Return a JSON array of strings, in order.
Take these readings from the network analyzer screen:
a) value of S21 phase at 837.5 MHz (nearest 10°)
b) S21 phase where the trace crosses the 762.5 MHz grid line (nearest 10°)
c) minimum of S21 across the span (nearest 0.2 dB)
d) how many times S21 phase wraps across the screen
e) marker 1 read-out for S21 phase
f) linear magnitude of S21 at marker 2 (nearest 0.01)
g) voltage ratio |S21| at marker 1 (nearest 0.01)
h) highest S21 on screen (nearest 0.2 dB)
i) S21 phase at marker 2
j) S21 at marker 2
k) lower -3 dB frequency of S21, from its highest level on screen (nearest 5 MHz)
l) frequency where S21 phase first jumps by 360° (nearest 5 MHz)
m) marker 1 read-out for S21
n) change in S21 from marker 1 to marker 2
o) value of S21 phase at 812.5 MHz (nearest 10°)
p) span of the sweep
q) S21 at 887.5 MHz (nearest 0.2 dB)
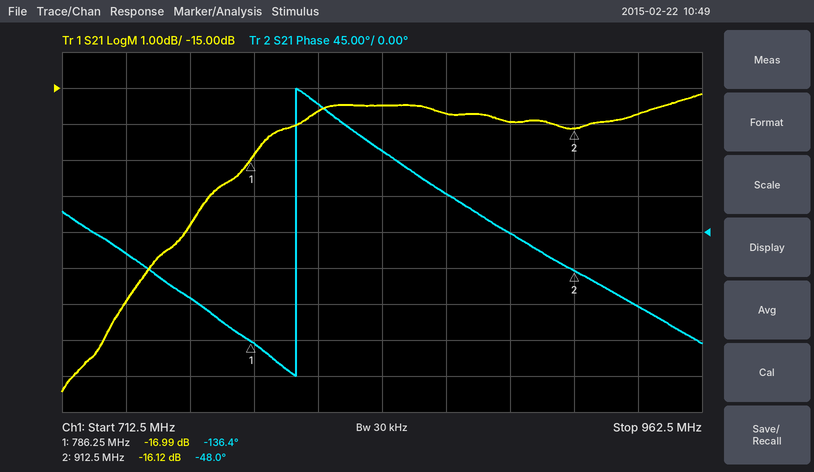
["100°", "-80°", "-23.4 dB", "1", "-136.4°", "0.16", "0.14", "-15.2 dB", "-48.0°", "-16.12 dB", "770 MHz", "805 MHz", "-16.99 dB", "0.87 dB", "160°", "250 MHz", "-16.0 dB"]
